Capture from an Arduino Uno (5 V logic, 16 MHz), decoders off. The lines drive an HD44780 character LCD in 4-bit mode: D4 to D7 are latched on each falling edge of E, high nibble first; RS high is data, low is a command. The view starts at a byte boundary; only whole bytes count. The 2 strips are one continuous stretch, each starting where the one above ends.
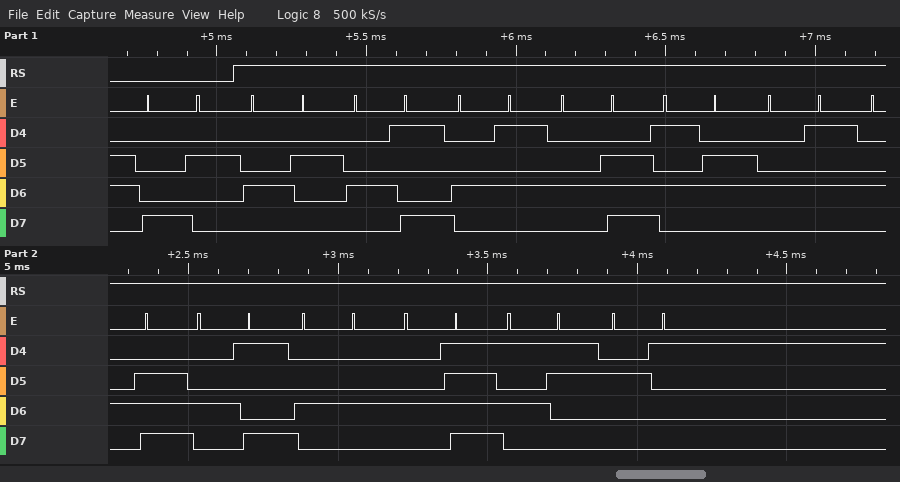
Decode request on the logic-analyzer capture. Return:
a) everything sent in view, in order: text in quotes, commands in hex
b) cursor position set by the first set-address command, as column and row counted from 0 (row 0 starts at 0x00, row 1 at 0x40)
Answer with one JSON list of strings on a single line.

["0x82 \"BIENVENIDOS!\"", "column 2, row 0"]
